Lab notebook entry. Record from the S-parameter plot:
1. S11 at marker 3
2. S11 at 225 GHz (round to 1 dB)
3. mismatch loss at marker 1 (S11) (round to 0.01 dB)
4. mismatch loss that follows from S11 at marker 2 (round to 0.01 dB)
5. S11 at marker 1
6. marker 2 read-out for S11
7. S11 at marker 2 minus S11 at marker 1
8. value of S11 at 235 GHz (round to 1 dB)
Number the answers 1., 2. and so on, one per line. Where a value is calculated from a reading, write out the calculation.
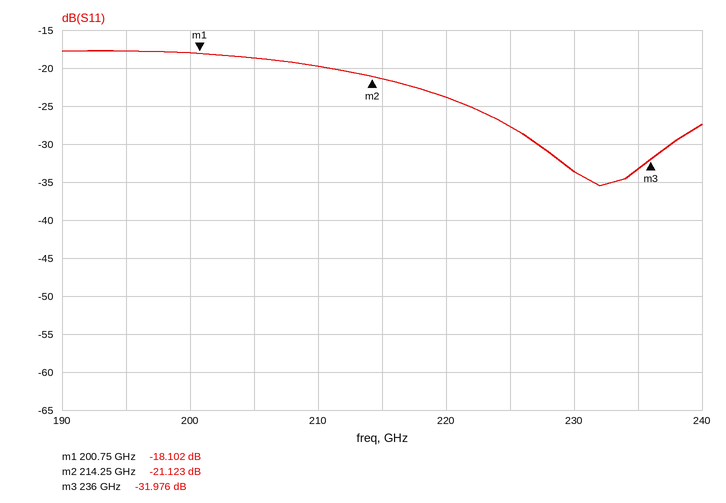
1. -31.976 dB
2. -28 dB
3. −10 log10(1 − 10^(-18.102/10)) ≈ 0.07 dB
4. −10 log10(1 − 10^(-21.123/10)) ≈ 0.03 dB
5. -18.102 dB
6. -21.123 dB
7. -21.123 − (-18.102) = -3.021 dB
8. -33 dB
